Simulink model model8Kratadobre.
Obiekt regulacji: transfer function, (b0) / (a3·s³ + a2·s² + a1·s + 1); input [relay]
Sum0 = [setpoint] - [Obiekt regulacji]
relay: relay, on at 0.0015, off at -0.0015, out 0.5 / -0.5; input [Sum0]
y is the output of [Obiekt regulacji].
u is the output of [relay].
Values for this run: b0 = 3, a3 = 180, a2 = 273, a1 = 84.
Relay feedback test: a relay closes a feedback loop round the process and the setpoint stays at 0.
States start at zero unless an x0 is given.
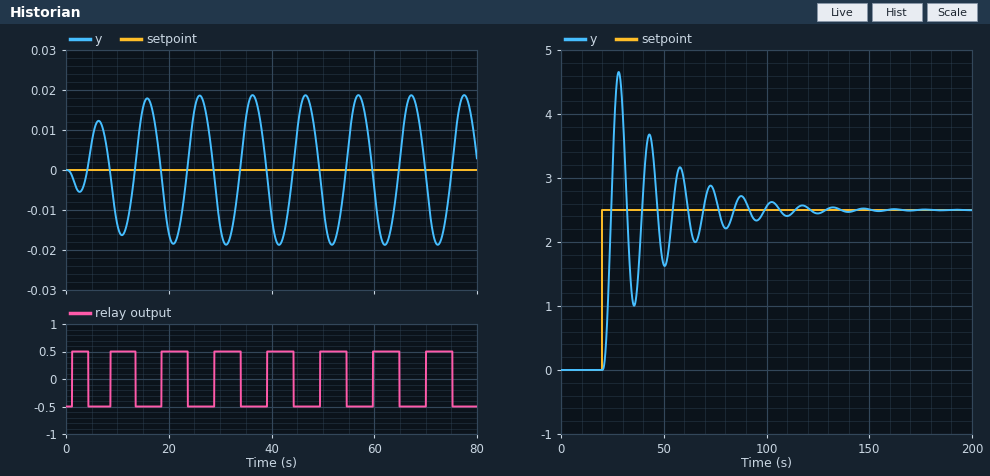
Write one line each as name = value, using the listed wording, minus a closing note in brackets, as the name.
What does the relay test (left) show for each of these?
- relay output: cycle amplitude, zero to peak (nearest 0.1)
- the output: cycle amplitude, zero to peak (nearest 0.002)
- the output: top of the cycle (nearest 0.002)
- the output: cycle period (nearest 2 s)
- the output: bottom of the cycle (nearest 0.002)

relay output: cycle amplitude, zero to peak = 0.5
the output: cycle amplitude, zero to peak = 0.018
the output: top of the cycle = 0.018
the output: cycle period = 10 s
the output: bottom of the cycle = -0.018
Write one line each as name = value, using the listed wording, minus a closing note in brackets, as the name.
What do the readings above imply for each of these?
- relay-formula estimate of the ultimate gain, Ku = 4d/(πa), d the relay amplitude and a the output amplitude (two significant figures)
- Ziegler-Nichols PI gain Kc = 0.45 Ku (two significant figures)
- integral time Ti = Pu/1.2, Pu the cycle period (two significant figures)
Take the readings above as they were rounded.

relay-formula estimate of the ultimate gain, Ku = 4d/(πa), d the relay amplitude and a the output amplitude = 35
Ziegler-Nichols PI gain Kc = 0.45 Ku = 16
integral time Ti = Pu/1.2, Pu the cycle period = 8.3 s
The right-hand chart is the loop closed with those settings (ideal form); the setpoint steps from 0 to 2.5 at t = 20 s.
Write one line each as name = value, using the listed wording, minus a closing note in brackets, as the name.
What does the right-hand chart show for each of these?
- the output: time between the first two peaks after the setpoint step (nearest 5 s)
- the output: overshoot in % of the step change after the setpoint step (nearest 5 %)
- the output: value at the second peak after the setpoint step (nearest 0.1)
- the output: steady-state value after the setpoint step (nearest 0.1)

the output: time between the first two peaks after the setpoint step = 15 s
the output: overshoot in % of the step change after the setpoint step = 85 %
the output: value at the second peak after the setpoint step = 3.7
the output: steady-state value after the setpoint step = 2.5
